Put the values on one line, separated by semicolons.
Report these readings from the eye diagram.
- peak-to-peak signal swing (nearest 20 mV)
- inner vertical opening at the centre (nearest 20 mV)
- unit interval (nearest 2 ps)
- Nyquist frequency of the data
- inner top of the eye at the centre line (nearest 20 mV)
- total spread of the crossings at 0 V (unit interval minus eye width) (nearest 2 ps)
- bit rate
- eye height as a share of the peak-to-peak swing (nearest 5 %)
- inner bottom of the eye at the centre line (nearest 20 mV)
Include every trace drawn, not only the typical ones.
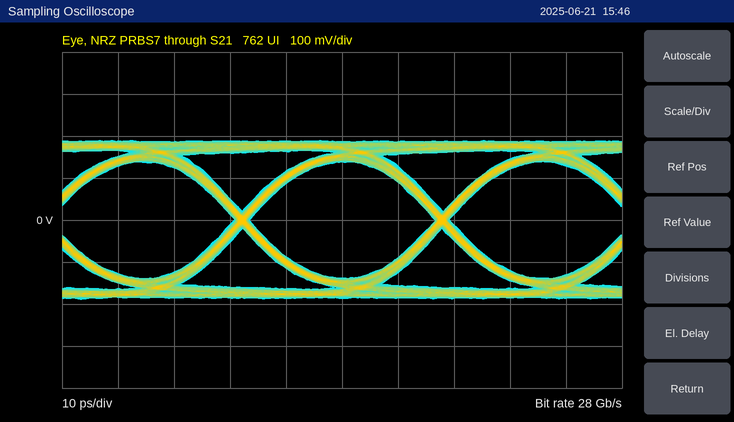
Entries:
380 mV; 280 mV; 36 ps; 14 GHz; 140 mV; 2 ps; 28 Gb/s; 75 %; -140 mV
